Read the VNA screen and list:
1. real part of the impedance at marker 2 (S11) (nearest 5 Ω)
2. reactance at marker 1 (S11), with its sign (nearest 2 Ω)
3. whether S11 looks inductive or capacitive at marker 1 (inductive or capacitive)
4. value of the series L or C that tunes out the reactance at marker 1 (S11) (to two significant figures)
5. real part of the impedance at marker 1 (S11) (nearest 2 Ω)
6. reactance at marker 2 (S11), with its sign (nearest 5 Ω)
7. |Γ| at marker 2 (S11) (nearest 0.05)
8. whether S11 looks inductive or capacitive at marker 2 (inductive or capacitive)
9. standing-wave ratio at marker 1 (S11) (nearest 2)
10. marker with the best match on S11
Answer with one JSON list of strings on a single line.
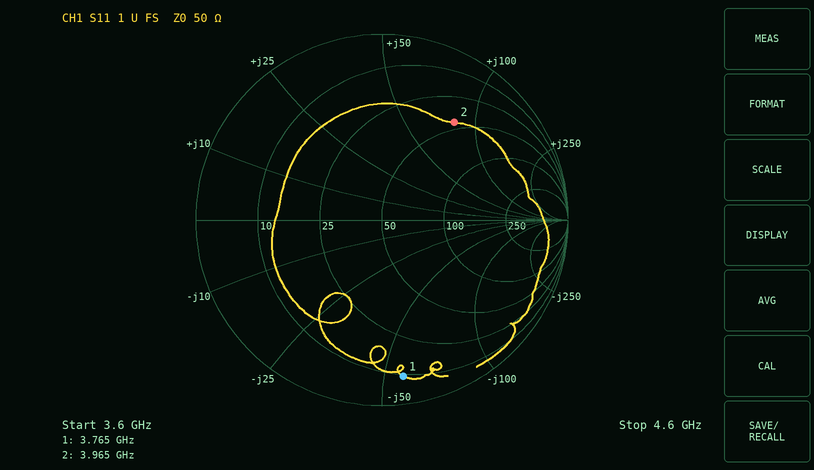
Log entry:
["45 Ω", "-56 Ω", "capacitive", "2.4 nH", "10 Ω", "+80 Ω", "0.65", "inductive", "12", "marker 2"]
